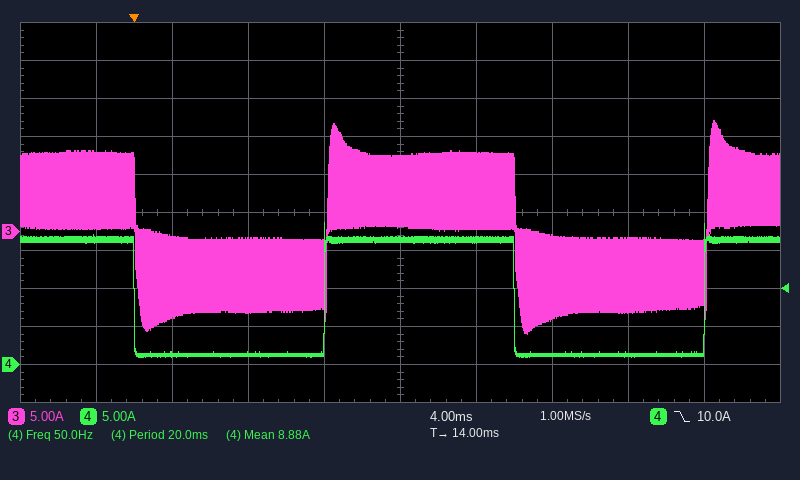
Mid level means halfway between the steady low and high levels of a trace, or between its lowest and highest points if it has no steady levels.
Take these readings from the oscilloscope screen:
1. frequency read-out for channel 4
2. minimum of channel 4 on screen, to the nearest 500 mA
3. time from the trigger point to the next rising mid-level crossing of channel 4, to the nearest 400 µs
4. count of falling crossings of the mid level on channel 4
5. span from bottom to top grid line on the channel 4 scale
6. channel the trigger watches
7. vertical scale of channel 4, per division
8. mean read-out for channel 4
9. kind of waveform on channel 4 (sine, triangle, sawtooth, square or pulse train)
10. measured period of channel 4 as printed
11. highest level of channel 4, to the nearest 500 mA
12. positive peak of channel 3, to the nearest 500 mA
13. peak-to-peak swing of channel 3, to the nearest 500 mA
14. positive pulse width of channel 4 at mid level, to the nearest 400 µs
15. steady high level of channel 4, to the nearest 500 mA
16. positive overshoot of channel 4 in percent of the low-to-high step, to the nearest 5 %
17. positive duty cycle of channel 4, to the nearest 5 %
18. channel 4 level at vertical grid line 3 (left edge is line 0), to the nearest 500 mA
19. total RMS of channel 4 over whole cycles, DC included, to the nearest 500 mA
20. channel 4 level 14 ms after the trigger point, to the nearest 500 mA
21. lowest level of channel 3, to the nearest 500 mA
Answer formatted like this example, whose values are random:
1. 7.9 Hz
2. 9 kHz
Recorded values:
1. 50.0 Hz
2. 1.0 A
3. 10.0 ms
4. 2
5. 50 A
6. channel 4
7. 5 A
8. 8.88 A
9. square
10. 20.0 ms
11. 18.5 A
12. 14.5 A
13. 28.0 A
14. 10.0 ms
15. 16.5 A
16. 15 %
17. 50 %
18. 1.5 A
19. 11.5 A
20. 16.5 A
21. -13.5 A
